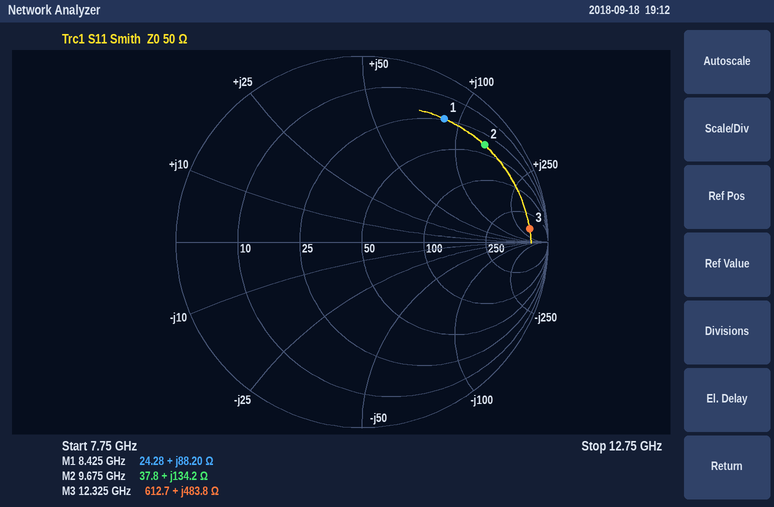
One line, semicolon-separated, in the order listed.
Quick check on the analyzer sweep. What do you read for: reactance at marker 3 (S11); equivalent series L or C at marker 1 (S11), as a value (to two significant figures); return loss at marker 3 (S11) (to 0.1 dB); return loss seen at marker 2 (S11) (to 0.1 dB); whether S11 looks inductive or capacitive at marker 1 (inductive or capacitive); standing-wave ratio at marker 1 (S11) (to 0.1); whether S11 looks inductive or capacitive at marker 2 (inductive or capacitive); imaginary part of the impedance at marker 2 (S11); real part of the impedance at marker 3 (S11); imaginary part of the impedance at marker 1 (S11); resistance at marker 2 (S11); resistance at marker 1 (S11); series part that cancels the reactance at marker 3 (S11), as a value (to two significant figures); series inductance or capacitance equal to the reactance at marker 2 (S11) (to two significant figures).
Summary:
+483.8 Ω; 1.7 nH; 0.9 dB; 1.5 dB; inductive; 8.8; inductive; +134.2 Ω; 612.7 Ω; +88.20 Ω; 37.8 Ω; 24.28 Ω; 27 fF; 2.2 nH
